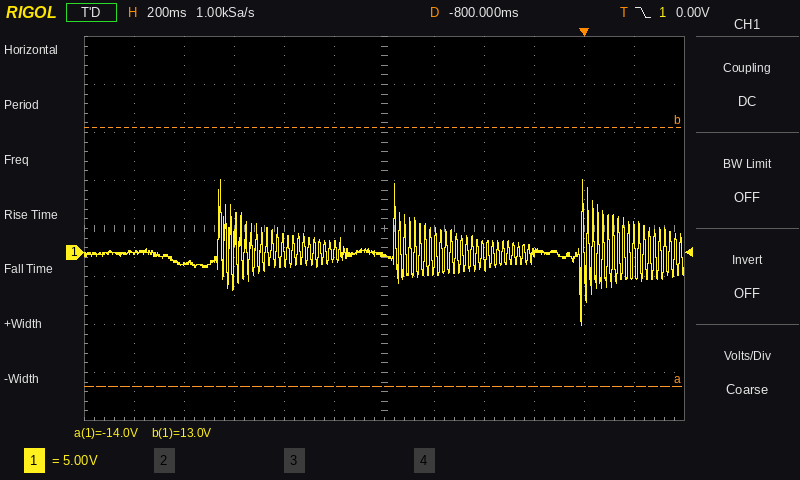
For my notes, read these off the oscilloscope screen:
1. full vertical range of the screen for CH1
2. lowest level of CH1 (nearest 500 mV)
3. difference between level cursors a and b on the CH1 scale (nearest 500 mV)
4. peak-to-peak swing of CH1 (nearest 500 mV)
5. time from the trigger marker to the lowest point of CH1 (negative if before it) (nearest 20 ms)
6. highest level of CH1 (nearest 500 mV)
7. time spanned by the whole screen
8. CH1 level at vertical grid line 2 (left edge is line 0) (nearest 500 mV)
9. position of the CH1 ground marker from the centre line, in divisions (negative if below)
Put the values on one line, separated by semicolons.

40 V; -7.5 V; 27.0 V; 15.0 V; -20 ms; 7.5 V; 2.4 s; -1.0 V; -0.5 div
